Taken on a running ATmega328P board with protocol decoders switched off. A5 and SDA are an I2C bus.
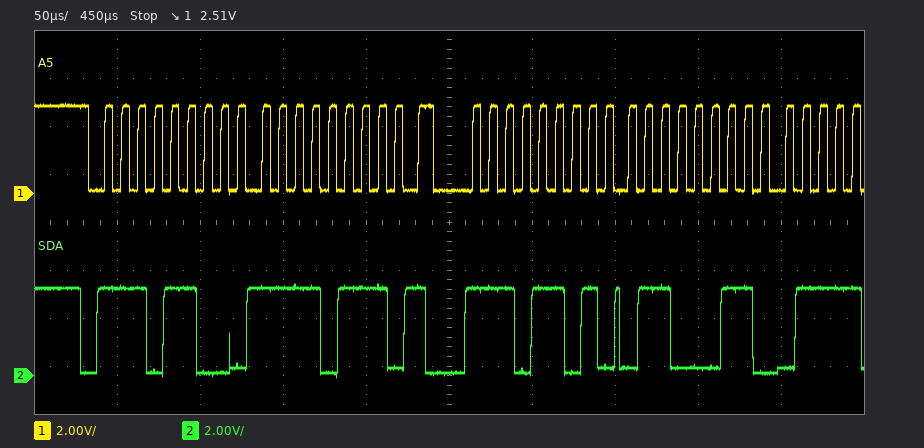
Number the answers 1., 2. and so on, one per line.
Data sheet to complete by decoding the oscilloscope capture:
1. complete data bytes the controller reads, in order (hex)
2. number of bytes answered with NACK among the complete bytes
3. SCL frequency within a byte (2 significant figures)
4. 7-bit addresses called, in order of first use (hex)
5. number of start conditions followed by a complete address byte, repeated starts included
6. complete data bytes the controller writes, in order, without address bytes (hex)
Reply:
1. 63
2. 0
3. 100 kHz
4. 0x76
5. 2
6. F7
